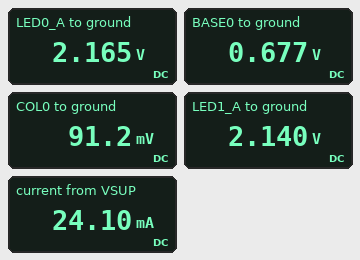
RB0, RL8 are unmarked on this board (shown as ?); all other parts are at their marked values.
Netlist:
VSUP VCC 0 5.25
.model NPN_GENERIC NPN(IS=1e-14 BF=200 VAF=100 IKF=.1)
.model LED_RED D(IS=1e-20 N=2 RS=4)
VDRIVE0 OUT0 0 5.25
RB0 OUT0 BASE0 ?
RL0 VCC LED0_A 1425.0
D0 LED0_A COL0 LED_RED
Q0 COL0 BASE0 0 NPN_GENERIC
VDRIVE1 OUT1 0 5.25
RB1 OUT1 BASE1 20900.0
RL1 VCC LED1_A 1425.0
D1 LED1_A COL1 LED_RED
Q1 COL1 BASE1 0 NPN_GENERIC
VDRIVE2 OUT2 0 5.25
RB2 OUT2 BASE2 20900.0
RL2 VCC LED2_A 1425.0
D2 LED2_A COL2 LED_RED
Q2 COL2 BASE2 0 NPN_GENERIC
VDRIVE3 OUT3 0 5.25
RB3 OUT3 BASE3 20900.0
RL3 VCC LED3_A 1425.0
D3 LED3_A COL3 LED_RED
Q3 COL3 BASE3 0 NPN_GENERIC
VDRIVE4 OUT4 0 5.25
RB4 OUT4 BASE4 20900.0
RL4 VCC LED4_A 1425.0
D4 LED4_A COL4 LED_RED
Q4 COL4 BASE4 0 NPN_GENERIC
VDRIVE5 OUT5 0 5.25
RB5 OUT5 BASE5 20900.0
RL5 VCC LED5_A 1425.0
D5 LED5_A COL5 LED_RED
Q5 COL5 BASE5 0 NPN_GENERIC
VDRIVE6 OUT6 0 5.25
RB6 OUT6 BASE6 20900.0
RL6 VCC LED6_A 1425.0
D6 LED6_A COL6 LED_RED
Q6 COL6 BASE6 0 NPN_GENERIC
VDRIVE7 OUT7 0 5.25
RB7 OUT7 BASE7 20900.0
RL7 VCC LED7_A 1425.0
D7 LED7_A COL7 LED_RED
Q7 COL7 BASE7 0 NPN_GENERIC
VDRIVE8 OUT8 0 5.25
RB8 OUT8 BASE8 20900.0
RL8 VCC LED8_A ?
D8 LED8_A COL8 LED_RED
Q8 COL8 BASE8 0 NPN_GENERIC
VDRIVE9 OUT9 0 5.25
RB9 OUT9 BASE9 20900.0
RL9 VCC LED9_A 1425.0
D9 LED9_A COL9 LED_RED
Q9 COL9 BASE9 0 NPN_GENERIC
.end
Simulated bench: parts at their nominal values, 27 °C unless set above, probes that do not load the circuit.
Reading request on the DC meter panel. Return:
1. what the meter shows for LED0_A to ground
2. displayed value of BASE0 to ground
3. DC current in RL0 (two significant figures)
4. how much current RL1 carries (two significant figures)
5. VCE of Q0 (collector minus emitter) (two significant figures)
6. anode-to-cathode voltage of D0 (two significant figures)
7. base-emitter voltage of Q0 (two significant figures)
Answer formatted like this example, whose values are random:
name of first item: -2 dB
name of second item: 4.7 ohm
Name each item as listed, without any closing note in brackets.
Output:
what the meter shows for LED0_A to ground: 2.165 V
displayed value of BASE0 to ground: 0.677 V
DC current in RL0: 2.2 mA
how much current RL1 carries: 2.2 mA
VCE of Q0 (collector minus emitter): 91 mV
anode-to-cathode voltage of D0: 2.1 V
base-emitter voltage of Q0: 680 mV
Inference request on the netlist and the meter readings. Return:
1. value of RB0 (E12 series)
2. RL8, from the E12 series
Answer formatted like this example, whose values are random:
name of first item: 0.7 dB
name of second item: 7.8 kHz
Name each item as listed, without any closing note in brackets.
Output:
value of RB0: 56 kΩ
RL8, from the E12 series: 680 Ω
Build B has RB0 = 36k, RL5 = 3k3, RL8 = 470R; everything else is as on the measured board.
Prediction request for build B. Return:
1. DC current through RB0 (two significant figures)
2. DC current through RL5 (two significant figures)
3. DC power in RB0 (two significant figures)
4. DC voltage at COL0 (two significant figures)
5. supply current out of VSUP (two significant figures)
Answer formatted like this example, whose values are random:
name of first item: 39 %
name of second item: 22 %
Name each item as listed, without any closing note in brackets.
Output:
DC current through RB0: 130 µA
DC current through RL5: 960 µA
DC power in RB0: 580 µW
DC voltage at COL0: 79 mV
supply current out of VSUP: 25 mA
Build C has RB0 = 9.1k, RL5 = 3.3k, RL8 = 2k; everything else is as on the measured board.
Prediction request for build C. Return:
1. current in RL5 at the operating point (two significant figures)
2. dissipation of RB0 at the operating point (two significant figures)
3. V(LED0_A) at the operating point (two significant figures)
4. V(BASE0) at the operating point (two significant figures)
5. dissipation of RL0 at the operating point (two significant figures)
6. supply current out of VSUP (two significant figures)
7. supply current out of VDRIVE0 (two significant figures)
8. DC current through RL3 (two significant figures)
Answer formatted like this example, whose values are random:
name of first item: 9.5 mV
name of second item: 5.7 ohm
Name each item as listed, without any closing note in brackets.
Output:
current in RL5 at the operating point: 960 µA
dissipation of RB0 at the operating point: 2.3 mW
V(LED0_A) at the operating point: 2.1 V
V(BASE0) at the operating point: 690 mV
dissipation of RL0 at the operating point: 6.9 mW
supply current out of VSUP: 20 mA
supply current out of VDRIVE0: 500 µA
DC current through RL3: 2.2 mA
